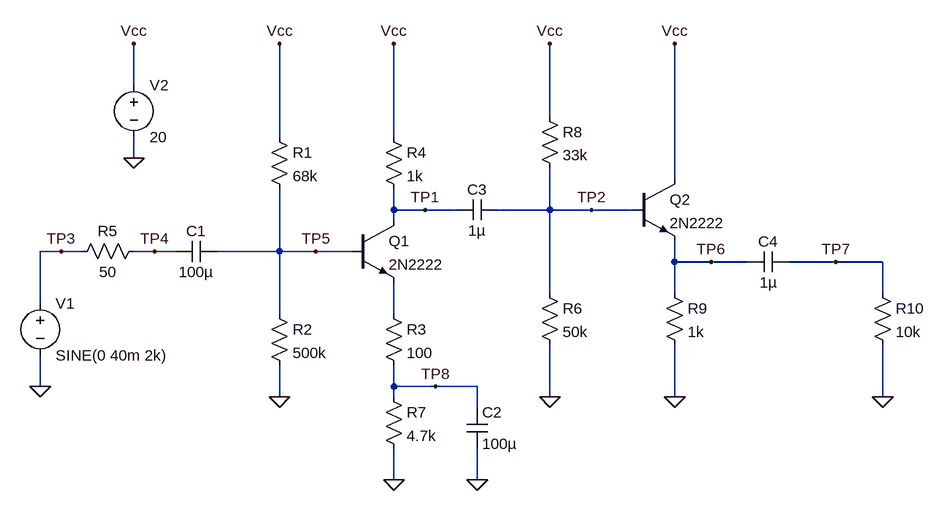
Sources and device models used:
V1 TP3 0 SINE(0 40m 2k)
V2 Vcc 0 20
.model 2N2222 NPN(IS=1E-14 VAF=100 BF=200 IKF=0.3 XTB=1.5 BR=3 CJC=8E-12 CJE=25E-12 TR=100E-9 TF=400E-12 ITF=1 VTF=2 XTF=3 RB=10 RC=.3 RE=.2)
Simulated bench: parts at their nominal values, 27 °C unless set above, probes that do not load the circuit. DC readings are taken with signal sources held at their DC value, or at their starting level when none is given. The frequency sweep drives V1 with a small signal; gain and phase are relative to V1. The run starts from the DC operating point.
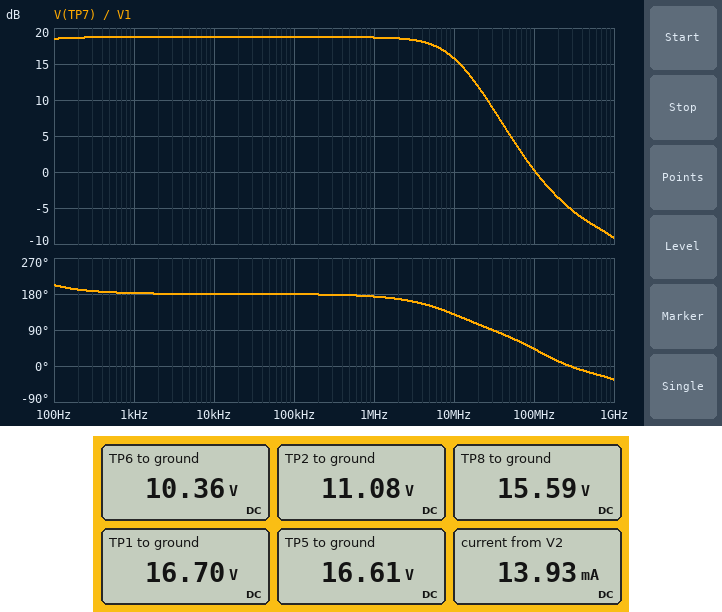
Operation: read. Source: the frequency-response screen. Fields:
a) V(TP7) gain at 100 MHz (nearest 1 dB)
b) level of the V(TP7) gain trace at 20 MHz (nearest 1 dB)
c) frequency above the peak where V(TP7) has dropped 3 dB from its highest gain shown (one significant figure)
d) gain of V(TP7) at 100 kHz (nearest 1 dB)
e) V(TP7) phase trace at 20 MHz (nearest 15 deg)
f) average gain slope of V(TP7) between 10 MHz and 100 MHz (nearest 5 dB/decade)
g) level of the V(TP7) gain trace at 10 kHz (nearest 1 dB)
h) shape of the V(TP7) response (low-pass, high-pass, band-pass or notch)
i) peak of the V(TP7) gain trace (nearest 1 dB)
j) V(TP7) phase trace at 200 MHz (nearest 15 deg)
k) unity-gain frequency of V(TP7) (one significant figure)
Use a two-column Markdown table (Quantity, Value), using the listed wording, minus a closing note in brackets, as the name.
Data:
| Quantity | Value |
|---|---|
| V(TP7) gain at 100 MHz | 0 dB |
| level of the V(TP7) gain trace at 20 MHz | 12 dB |
| frequency above the peak where V(TP7) has dropped 3 dB from its highest gain shown | 10 MHz |
| gain of V(TP7) at 100 kHz | 19 dB |
| V(TP7) phase trace at 20 MHz | 105 deg |
| average gain slope of V(TP7) between 10 MHz and 100 MHz | -15 dB/decade |
| level of the V(TP7) gain trace at 10 kHz | 19 dB |
| shape of the V(TP7) response | low-pass |
| peak of the V(TP7) gain trace | 19 dB |
| V(TP7) phase trace at 200 MHz | 15 deg |
| unity-gain frequency of V(TP7) | 100 MHz |
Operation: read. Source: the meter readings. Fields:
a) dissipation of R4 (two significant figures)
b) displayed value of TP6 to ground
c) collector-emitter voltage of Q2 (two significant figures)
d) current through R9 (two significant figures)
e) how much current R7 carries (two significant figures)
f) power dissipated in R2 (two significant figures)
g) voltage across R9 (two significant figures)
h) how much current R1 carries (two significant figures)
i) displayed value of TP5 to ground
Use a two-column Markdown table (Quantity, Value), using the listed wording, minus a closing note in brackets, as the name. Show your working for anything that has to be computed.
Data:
| Quantity | Value |
|---|---|
| dissipation of R4 | (20 V - 16.7 V)^2 / 1 kΩ = 11 mW |
| displayed value of TP6 to ground | 10.36 V |
| collector-emitter voltage of Q2 | 20 V - 10.36 V = 9.6 V |
| current through R9 | (10.36 V) / 1 kΩ = 10 mA |
| how much current R7 carries | (15.59 V) / 4.7 kΩ = 3.3 mA |
| power dissipated in R2 | (16.61 V)^2 / 500 kΩ = 550 µW |
| voltage across R9 | 10.36 V = 10 V |
| how much current R1 carries | (20 V - 16.61 V) / 68 kΩ = 50 µA |
| displayed value of TP5 to ground | 16.61 V |
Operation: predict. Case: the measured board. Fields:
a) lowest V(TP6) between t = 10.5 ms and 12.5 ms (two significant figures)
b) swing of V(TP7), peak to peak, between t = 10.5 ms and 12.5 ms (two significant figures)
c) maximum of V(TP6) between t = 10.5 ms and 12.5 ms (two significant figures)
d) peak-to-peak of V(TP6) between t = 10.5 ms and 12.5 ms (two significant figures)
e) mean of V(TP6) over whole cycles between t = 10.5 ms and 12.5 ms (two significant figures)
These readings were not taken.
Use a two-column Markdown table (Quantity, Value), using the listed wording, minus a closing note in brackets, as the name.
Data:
| Quantity | Value |
|---|---|
| lowest V(TP6) between t = 10.5 ms and 12.5 ms | 10 V |
| swing of V(TP7), peak to peak, between t = 10.5 ms and 12.5 ms | 690 mV |
| maximum of V(TP6) between t = 10.5 ms and 12.5 ms | 11 V |
| peak-to-peak of V(TP6) between t = 10.5 ms and 12.5 ms | 690 mV |
| mean of V(TP6) over whole cycles between t = 10.5 ms and 12.5 ms | 10 V |
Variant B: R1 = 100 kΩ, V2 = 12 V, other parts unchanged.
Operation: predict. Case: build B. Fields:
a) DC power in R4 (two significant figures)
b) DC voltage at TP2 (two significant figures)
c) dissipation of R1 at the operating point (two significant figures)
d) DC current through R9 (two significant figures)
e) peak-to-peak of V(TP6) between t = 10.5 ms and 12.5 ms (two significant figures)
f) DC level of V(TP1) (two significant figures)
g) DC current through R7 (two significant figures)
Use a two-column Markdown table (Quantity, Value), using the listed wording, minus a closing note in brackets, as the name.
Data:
| Quantity | Value |
|---|---|
| DC power in R4 | 3.2 mW |
| DC voltage at TP2 | 6.7 V |
| dissipation of R1 at the operating point | 75 µW |
| DC current through R9 | 6.0 mA |
| peak-to-peak of V(TP6) between t = 10.5 ms and 12.5 ms | 650 mV |
| DC level of V(TP1) | 10 V |
| DC current through R7 | 1.8 mA |
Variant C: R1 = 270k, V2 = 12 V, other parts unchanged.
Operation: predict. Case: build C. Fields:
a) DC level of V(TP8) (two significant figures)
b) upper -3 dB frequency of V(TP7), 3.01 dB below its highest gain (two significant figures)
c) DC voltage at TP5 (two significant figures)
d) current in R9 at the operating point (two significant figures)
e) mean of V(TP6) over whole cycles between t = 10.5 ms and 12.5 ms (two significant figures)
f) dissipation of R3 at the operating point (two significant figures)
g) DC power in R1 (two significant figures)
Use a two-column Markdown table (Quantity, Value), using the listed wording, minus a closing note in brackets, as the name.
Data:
| Quantity | Value |
|---|---|
| DC level of V(TP8) | 5.9 V |
| upper -3 dB frequency of V(TP7), 3.01 dB below its highest gain | 14 MHz |
| DC voltage at TP5 | 6.7 V |
| current in R9 at the operating point | 6.0 mA |
| mean of V(TP6) over whole cycles between t = 10.5 ms and 12.5 ms | 6.0 V |
| dissipation of R3 at the operating point | 160 µW |
| DC power in R1 | 100 µW |
